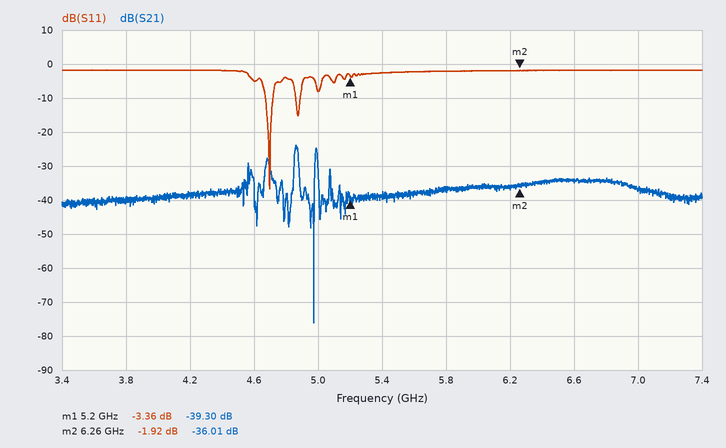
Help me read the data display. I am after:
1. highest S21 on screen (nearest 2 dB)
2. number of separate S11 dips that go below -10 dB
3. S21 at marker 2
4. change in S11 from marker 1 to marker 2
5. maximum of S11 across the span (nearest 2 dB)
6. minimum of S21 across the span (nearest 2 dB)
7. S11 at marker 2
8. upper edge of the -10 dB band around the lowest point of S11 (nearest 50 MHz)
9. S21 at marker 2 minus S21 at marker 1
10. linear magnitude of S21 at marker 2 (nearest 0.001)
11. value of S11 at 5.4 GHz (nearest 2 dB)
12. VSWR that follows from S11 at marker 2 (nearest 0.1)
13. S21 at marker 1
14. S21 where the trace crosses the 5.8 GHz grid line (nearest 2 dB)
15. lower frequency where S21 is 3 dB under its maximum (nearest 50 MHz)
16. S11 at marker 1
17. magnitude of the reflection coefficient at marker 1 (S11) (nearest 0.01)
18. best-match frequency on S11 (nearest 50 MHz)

-24 dB
2
-36.01 dB
1.44 dB
-2 dB
-76 dB
-1.92 dB
4.70 GHz
3.29 dB
0.016
-2 dB
9.1
-39.30 dB
-36 dB
4.85 GHz
-3.36 dB
0.68
4.70 GHz
